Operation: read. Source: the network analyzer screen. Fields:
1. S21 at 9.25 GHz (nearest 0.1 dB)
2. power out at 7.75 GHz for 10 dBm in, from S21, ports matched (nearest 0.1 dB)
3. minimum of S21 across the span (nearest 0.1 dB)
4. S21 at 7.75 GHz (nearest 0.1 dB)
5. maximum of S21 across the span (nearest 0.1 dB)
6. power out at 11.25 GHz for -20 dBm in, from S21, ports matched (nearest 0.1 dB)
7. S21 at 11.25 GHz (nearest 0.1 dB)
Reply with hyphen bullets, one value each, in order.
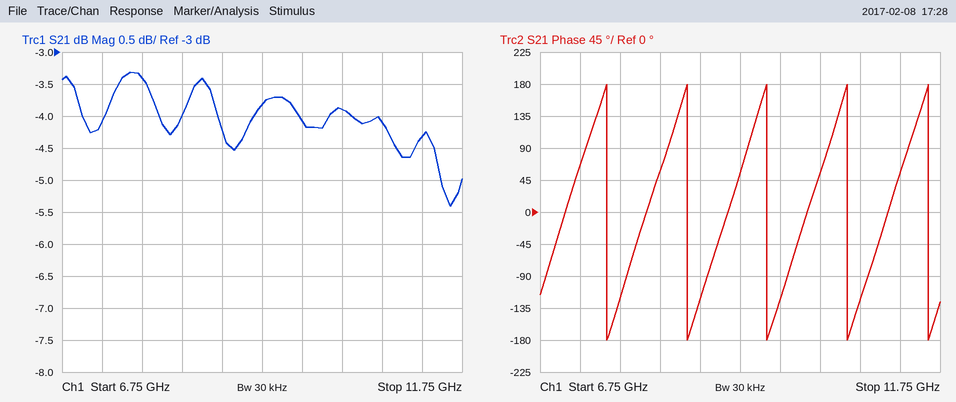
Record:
- -3.8 dB
- 6.6 dBm
- -5.4 dB
- -3.4 dB
- -3.3 dB
- -24.3 dBm
- -4.3 dB
